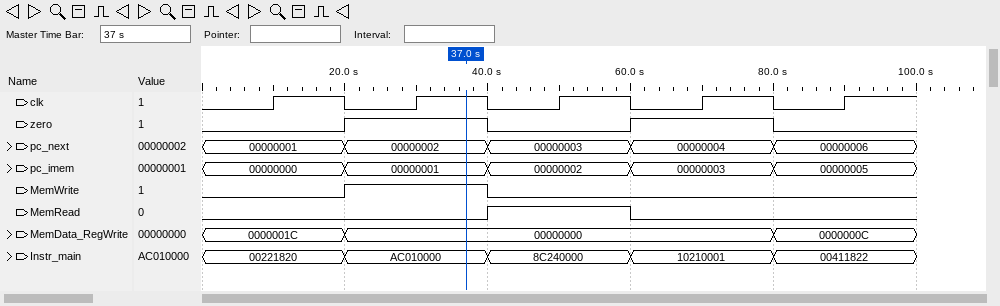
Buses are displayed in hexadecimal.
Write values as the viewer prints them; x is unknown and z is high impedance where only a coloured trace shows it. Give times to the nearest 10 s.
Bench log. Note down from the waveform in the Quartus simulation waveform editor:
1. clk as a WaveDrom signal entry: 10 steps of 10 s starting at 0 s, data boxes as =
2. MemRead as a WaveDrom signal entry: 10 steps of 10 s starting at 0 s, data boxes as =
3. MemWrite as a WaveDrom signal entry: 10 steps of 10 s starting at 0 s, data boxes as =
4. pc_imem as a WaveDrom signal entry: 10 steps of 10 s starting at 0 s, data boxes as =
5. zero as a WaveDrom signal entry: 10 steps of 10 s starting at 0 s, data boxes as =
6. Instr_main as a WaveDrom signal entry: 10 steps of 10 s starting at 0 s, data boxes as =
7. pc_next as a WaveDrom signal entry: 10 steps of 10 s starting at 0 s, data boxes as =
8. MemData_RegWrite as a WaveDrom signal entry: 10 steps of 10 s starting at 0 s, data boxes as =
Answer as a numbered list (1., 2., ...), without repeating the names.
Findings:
1. {name: 'clk', wave: '0101010101'}
2. {name: 'MemRead', wave: '0...1.0...'}
3. {name: 'MemWrite', wave: '0.1.0.....'}
4. {name: 'pc_imem', wave: '=.=.=.=.=.', data: '00000000 00000001 00000002 00000003 00000005'}
5. {name: 'zero', wave: '0.1.0.1.0.'}
6. {name: 'Instr_main', wave: '=.=.=.=.=.', data: '00221820 AC010000 8C240000 10210001 00411822'}
7. {name: 'pc_next', wave: '=.=.=.=.=.', data: '00000001 00000002 00000003 00000004 00000006'}
8. {name: 'MemData_RegWrite', wave: '=.=.....=.', data: '0000001C 00000000 0000000C'}
